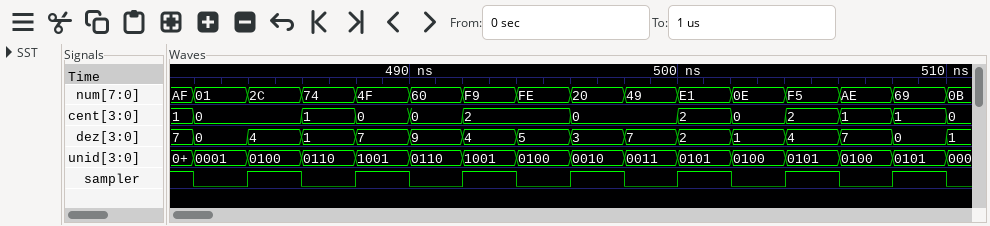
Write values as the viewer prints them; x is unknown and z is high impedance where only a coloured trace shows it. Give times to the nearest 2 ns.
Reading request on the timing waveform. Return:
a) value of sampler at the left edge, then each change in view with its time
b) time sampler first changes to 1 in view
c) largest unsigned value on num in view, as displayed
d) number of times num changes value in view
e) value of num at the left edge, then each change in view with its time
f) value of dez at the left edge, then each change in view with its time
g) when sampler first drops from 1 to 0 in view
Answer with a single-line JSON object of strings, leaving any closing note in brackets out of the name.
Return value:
{"value of sampler at the left edge, then each change in view with its time": "1, 0 at 482 ns, 1 at 484 ns, 0 at 486 ns, 1 at 488 ns, 0 at 490 ns, 1 at 492 ns, 0 at 494 ns, 1 at 496 ns, 0 at 498 ns, 1 at 500 ns, 0 at 502 ns, 1 at 504 ns, 0 at 506 ns, 1 at 508 ns, 0 at 510 ns", "time sampler first changes to 1 in view": "484 ns", "largest unsigned value on num in view, as displayed": "FE", "number of times num changes value in view": "15", "value of num at the left edge, then each change in view with its time": "AF, 01 at 482 ns, 2C at 484 ns, 74 at 486 ns, 4F at 488 ns, 60 at 490 ns, F9 at 492 ns, FE at 494 ns, 20 at 496 ns, 49 at 498 ns, E1 at 500 ns, 0E at 502 ns, F5 at 504 ns, AE at 506 ns, 69 at 508 ns, 0B at 510 ns", "value of dez at the left edge, then each change in view with its time": "7, 0 at 482 ns, 4 at 484 ns, 1 at 486 ns, 7 at 488 ns, 9 at 490 ns, 4 at 492 ns, 5 at 494 ns, 3 at 496 ns, 7 at 498 ns, 2 at 500 ns, 1 at 502 ns, 4 at 504 ns, 7 at 506 ns, 0 at 508 ns, 1 at 510 ns", "when sampler first drops from 1 to 0 in view": "482 ns"}
